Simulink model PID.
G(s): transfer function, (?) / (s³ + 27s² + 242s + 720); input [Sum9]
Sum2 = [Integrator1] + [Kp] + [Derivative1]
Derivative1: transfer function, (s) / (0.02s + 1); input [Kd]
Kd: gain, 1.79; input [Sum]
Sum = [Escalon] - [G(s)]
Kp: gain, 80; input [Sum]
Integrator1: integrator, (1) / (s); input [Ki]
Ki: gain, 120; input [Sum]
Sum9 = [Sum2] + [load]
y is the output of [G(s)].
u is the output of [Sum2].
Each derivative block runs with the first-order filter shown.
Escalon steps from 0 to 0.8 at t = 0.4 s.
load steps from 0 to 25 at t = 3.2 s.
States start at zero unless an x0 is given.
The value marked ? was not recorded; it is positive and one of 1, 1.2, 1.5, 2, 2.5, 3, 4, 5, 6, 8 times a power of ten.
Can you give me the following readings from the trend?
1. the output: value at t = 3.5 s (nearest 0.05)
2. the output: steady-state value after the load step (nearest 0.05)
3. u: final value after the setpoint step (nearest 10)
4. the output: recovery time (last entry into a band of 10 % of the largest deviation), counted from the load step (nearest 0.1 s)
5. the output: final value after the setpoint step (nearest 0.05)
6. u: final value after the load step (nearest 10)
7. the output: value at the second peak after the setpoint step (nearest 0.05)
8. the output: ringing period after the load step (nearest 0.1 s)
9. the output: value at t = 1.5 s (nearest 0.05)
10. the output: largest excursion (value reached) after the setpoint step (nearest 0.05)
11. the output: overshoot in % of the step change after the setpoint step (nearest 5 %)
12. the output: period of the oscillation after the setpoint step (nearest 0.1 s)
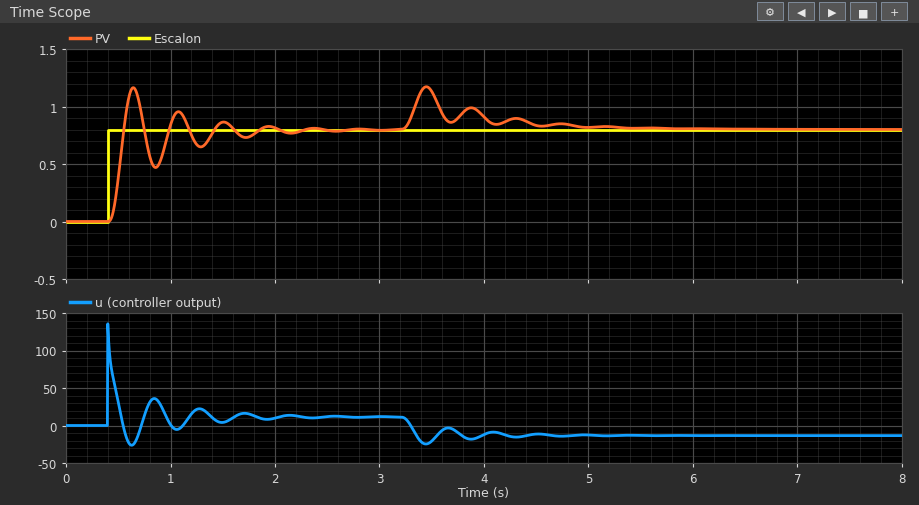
1.15
0.80
10
1.6 s
0.80
-10
0.95
0.4 s
0.85
1.15
45 %
0.4 s
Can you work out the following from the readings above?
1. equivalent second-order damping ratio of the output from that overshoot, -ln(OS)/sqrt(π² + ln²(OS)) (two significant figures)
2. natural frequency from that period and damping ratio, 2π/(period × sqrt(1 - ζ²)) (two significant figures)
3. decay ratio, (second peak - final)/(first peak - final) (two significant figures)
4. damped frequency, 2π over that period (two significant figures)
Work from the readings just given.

0.25
16 rad/s
0.43
16 rad/s
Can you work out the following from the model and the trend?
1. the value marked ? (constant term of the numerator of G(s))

50
